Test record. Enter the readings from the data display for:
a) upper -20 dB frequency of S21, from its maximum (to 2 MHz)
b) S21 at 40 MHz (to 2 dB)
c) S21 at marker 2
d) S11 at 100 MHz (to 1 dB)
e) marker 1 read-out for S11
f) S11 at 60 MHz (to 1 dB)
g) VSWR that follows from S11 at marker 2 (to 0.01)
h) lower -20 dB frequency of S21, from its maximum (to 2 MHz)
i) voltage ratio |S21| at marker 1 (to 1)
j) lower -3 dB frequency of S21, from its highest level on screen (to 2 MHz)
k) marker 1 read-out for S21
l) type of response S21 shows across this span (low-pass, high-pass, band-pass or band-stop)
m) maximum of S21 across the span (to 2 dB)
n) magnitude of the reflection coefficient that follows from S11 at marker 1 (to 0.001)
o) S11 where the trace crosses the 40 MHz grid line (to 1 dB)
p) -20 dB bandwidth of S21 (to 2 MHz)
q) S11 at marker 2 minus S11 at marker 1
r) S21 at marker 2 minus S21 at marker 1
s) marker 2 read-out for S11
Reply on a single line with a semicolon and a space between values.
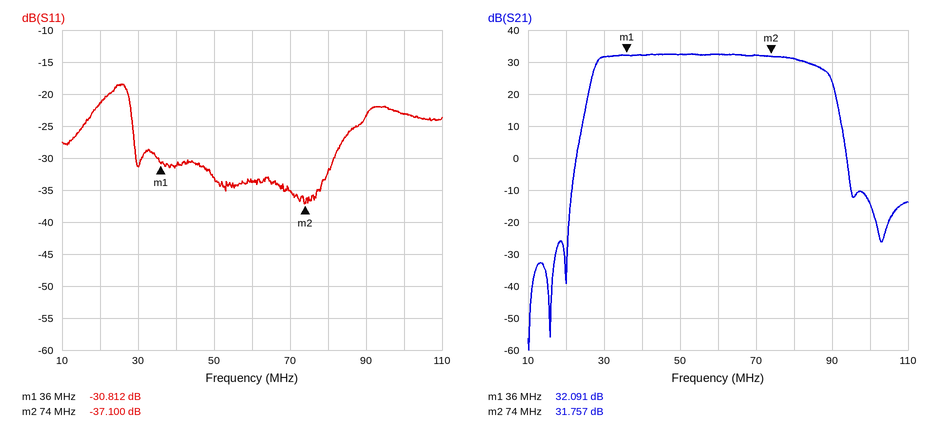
92 MHz; 32 dB; 31.757 dB; -23 dB; -30.812 dB; -34 dB; 1.03; 24 MHz; 40; 28 MHz; 32.091 dB; band-pass; 32 dB; 0.029; -31 dB; 68 MHz; -6.288 dB; -0.334 dB; -37.100 dB
